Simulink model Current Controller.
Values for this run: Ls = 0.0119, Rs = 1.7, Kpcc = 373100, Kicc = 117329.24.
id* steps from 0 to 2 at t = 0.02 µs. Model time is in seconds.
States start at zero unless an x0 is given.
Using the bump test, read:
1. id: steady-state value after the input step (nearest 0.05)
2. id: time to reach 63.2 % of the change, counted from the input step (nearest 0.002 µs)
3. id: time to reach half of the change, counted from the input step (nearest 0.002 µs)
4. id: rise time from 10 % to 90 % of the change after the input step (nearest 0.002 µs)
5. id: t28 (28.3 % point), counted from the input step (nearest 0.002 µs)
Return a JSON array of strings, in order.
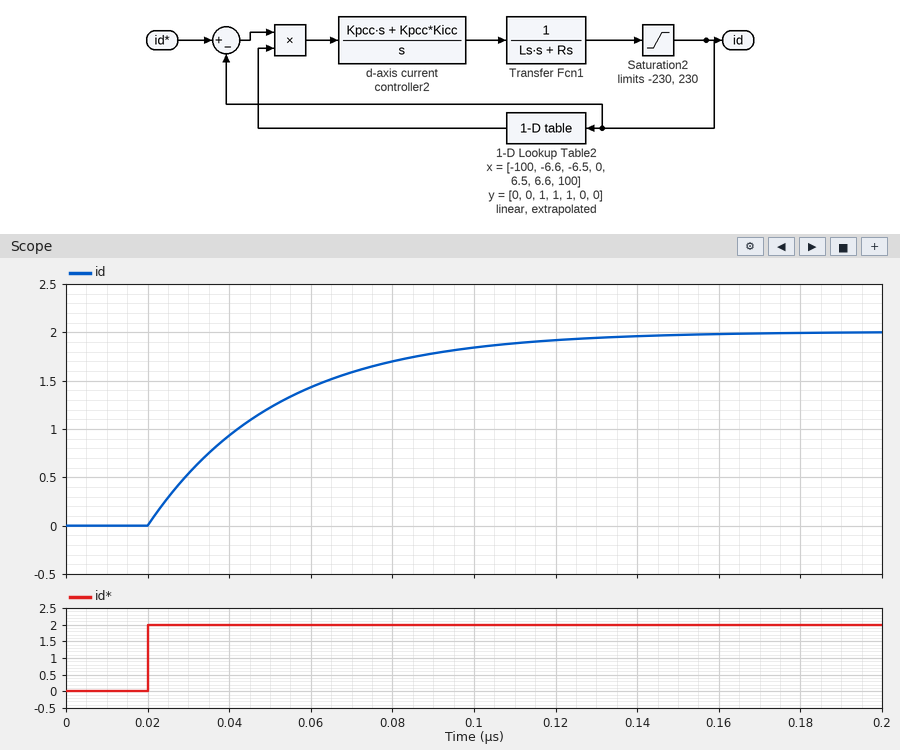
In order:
["2.00", "0.032 µs", "0.022 µs", "0.070 µs", "0.010 µs"]
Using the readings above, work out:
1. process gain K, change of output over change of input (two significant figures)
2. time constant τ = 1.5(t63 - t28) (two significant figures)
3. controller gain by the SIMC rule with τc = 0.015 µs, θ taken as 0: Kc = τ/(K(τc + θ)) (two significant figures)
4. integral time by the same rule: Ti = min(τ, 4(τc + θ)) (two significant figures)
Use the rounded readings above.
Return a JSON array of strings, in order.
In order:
["1.0", "0.033 µs", "2.2", "0.033 µs"]
